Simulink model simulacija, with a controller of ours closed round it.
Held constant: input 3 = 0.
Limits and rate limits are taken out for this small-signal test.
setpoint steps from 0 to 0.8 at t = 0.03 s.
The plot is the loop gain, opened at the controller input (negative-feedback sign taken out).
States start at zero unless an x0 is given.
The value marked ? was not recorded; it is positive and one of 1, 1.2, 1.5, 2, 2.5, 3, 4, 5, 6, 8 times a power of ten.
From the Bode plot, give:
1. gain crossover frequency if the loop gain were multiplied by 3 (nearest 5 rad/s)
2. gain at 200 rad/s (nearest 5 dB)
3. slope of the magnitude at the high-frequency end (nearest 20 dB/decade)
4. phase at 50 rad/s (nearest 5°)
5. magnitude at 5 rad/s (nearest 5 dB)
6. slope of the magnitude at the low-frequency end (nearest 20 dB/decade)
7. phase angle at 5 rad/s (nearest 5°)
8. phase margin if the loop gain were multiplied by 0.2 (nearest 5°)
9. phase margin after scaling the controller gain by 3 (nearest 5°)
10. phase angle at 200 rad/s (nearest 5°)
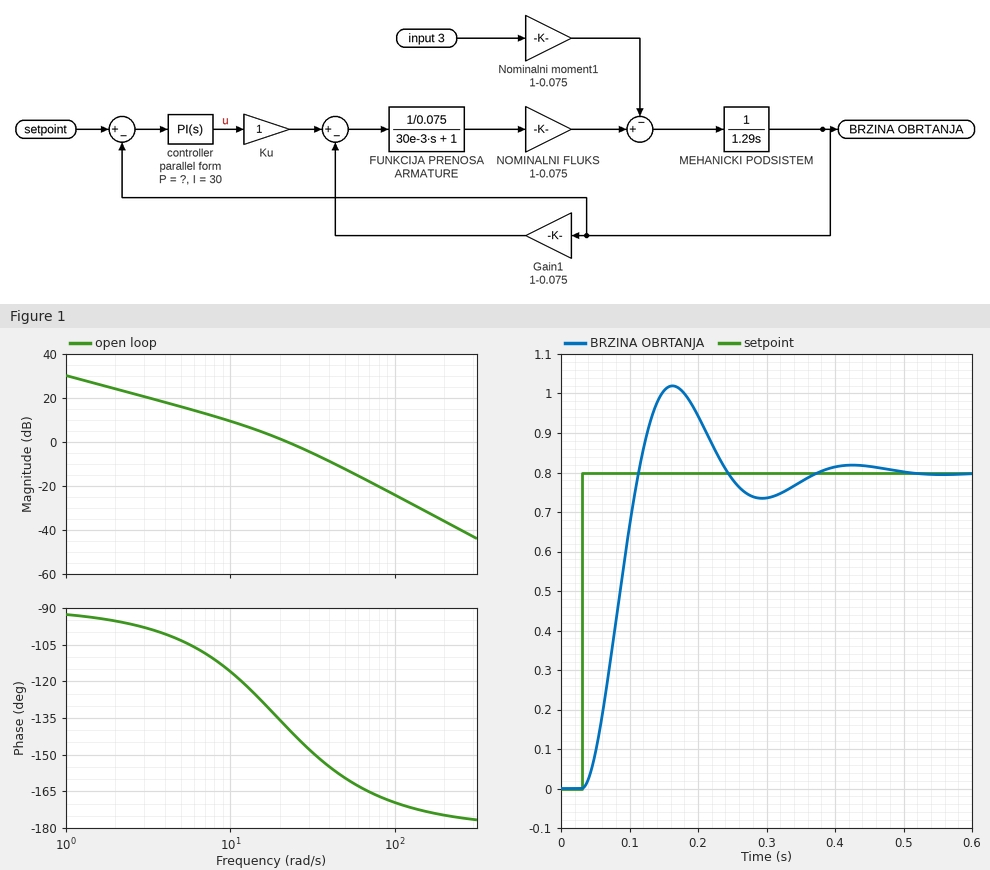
40 rad/s
-35 dB
-40 dB/decade
-160°
15 dB
-20 dB/decade
-105°
75°
25°
-175°
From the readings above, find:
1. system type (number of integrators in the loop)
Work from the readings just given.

1
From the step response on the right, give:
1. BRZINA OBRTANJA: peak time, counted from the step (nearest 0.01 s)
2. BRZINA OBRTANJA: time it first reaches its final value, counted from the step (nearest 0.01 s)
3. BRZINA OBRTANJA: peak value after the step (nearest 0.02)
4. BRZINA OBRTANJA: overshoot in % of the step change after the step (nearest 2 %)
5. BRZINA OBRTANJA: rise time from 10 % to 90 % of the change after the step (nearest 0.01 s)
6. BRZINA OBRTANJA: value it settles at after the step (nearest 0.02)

0.13 s
0.08 s
1.02
28 %
0.06 s
0.80
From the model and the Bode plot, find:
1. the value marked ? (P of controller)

2
